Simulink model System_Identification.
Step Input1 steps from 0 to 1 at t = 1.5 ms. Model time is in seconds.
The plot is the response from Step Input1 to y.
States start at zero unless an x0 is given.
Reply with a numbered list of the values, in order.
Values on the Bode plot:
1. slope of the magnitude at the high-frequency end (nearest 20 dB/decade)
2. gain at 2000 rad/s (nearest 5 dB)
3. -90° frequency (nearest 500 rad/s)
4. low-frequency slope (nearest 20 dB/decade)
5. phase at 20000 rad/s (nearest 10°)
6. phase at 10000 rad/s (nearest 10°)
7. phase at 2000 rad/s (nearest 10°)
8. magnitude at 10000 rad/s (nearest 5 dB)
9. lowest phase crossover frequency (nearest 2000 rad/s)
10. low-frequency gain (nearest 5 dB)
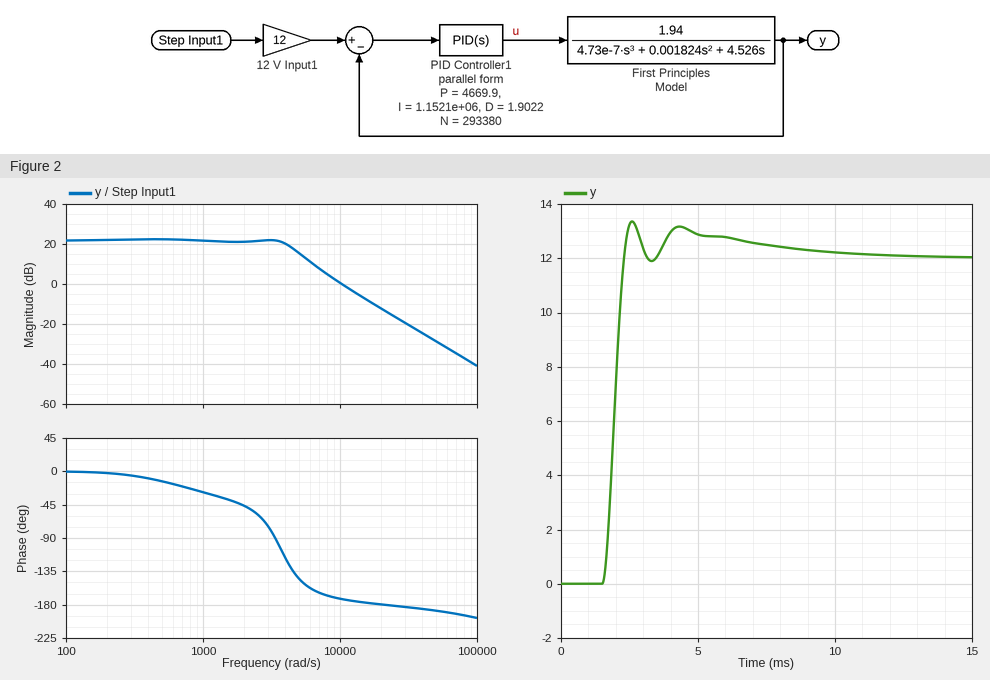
1. -40 dB/decade
2. 20 dB
3. 3500 rad/s
4. 0 dB/decade
5. -180°
6. -170°
7. -50°
8. 0 dB
9. 20000 rad/s
10. 20 dB
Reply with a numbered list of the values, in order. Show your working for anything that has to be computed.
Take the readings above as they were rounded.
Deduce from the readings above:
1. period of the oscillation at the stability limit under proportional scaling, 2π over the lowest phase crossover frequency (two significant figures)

1. 2π / 20000 = 0.00031 s
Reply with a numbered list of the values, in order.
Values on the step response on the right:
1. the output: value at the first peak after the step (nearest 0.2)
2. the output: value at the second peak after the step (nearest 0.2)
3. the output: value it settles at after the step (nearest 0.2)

1. 13.4
2. 13.2
3. 12.0
